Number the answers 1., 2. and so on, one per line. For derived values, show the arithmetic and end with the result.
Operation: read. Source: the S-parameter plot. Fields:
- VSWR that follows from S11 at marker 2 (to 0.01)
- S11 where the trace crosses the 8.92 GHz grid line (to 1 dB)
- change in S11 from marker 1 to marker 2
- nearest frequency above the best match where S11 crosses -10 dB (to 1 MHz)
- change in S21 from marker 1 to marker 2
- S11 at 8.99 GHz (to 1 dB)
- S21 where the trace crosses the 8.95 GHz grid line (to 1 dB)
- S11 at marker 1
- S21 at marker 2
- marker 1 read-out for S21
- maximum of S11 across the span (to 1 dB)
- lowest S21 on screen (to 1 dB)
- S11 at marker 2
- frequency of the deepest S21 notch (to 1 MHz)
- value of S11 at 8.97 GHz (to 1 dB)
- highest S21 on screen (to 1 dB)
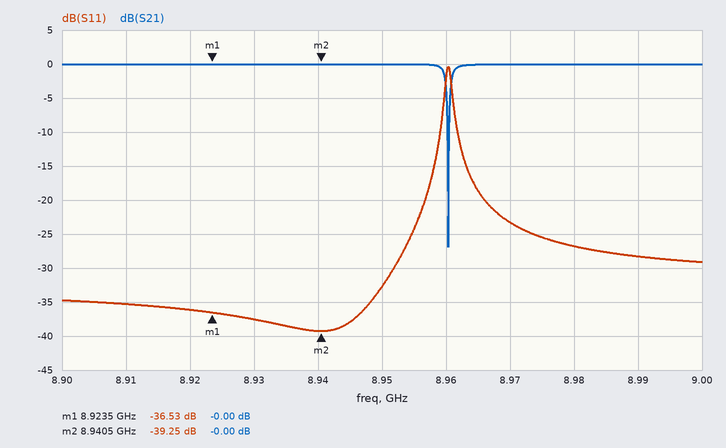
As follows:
1. (1 + 0.0109)/(1 − 0.0109) ≈ 1.02
2. -36 dB
3. -39.25 − (-36.53) = -2.72 dB
4. 8.959 GHz
5. -0 − (-0) = 0.00 dB
6. -28 dB
7. 0 dB
8. -36.53 dB
9. -0.00 dB
10. -0.00 dB
11. 0 dB
12. -27 dB
13. -39.25 dB
14. 8.960 GHz
15. -23 dB
16. 0 dB
